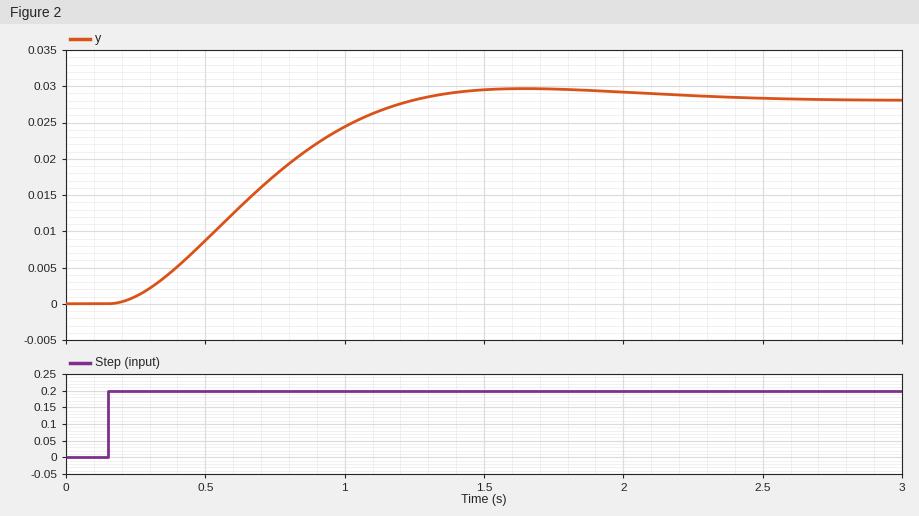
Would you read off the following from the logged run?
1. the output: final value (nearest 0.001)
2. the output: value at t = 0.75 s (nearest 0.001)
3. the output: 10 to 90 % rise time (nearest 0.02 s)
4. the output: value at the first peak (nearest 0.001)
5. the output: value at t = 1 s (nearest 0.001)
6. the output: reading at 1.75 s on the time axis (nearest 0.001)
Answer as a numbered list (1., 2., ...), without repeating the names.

1. 0.028
2. 0.018
3. 0.72 s
4. 0.030
5. 0.024
6. 0.030
